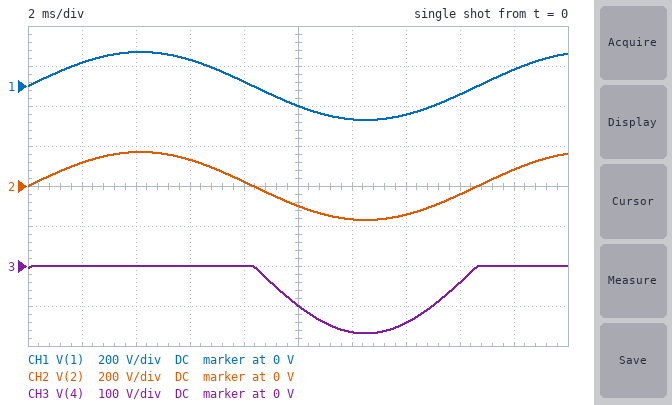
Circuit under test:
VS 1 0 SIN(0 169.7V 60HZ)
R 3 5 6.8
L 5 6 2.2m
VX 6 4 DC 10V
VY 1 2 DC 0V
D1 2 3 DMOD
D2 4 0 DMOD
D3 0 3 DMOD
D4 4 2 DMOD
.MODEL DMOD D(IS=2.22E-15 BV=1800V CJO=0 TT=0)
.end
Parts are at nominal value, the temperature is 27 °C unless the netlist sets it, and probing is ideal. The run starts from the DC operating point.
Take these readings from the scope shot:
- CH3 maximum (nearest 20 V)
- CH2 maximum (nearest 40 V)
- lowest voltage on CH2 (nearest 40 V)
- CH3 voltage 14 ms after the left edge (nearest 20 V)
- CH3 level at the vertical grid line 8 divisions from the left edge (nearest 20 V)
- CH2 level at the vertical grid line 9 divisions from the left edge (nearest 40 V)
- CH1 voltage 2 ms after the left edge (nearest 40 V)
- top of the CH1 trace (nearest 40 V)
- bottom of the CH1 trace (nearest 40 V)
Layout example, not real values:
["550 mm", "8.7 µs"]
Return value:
["0 V", "160 V", "-160 V", "-140 V", "-40 V", "80 V", "120 V", "160 V", "-160 V"]
